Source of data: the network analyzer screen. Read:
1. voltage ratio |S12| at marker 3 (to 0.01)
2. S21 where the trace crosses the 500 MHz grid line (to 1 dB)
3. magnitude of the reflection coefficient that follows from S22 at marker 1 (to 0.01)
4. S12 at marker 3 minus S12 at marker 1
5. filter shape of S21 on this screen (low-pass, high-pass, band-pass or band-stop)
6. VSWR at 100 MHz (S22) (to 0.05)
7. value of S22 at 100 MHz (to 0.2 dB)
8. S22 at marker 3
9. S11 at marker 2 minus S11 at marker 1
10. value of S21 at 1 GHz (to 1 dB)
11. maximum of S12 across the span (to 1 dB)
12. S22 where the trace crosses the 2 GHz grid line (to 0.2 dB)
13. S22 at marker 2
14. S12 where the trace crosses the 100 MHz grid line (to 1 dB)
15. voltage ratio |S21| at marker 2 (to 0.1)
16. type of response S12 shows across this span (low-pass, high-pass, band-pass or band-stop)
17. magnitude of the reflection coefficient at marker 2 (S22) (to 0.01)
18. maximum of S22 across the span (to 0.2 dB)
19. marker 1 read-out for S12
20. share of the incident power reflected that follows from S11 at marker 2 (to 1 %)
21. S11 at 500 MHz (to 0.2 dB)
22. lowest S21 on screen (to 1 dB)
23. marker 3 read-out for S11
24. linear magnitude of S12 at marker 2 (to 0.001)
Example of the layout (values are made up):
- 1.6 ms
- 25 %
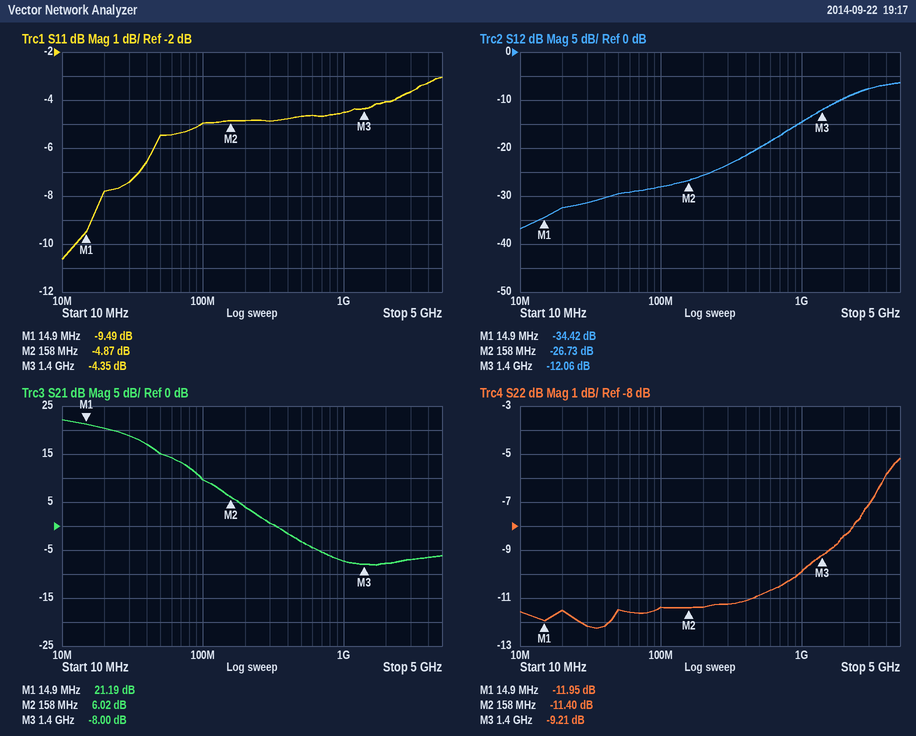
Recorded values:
- 0.25
- -3 dB
- 0.25
- 22.36 dB
- low-pass
- 1.75
- -11.4 dB
- -9.21 dB
- 4.62 dB
- -7 dB
- -6 dB
- -8.4 dB
- -11.40 dB
- -28 dB
- 2.0
- high-pass
- 0.27
- -5.2 dB
- -34.42 dB
- 33 %
- -4.6 dB
- -8 dB
- -4.35 dB
- 0.046
